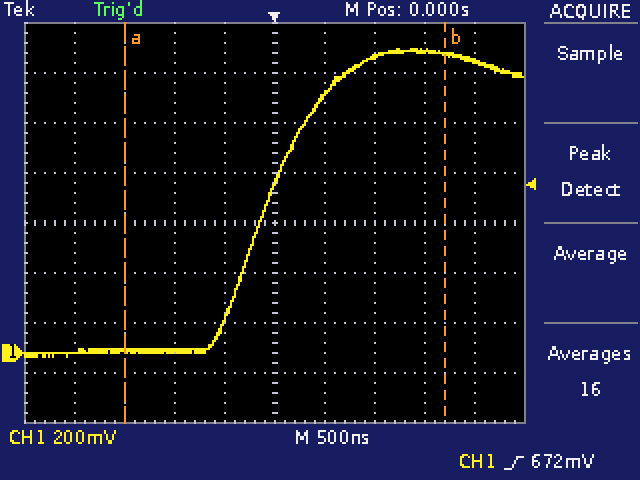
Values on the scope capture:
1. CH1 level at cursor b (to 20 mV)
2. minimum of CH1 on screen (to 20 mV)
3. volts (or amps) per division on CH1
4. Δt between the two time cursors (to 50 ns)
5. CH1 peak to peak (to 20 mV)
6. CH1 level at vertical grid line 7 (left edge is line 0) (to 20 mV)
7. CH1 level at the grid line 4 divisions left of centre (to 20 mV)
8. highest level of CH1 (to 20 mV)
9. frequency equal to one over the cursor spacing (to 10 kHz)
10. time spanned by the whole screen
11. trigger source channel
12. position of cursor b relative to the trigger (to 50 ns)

1.20 V
-20 mV
200 mV
3.20 µs
1.24 V
1.18 V
0 mV
1.22 V
310 kHz
5 µs
CH1
+1.70 µs
